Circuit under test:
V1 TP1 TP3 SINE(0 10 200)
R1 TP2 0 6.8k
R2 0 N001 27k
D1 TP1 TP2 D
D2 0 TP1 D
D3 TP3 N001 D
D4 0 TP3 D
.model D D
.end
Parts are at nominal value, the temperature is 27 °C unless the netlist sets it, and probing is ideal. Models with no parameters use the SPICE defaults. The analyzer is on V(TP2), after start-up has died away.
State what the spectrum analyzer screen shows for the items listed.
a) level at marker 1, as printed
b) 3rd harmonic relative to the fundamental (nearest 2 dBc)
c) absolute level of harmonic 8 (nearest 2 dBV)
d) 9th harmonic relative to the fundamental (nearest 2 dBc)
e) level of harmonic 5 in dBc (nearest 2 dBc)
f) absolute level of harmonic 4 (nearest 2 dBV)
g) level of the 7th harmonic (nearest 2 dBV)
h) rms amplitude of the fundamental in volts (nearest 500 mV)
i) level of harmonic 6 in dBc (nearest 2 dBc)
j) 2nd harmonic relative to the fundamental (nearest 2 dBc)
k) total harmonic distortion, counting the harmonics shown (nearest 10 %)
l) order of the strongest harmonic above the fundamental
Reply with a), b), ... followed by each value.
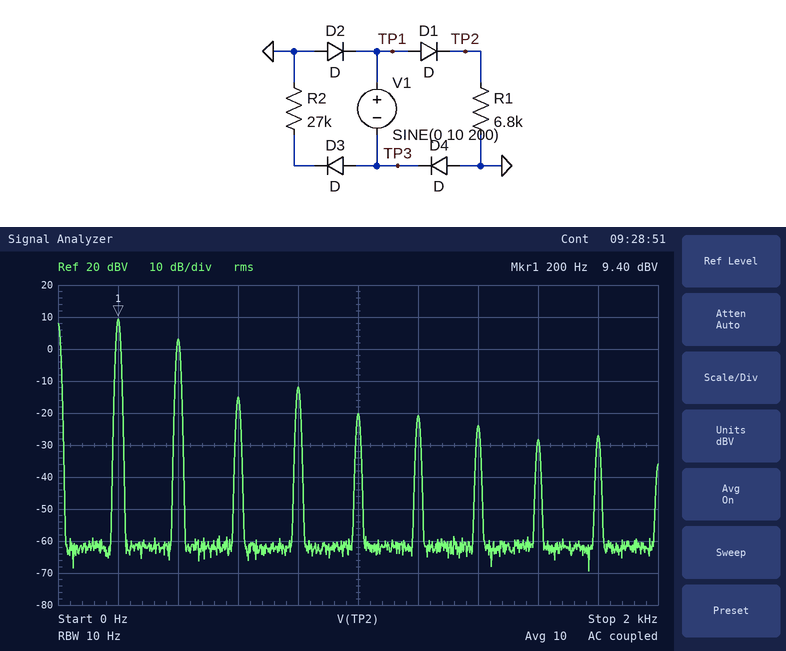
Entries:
a) 9.40 dBV
b) -24 dBc
c) -28 dBV
d) -36 dBc
e) -30 dBc
f) -12 dBV
g) -24 dBV
h) 3.0 V
i) -30 dBc
j) -6 dBc
k) 50 %
l) 2
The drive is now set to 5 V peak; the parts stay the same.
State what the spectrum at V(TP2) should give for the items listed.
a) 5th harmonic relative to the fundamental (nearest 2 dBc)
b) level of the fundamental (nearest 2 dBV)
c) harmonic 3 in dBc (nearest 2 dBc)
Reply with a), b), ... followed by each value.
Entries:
a) -24 dBc
b) 2 dBV
c) -18 dBc
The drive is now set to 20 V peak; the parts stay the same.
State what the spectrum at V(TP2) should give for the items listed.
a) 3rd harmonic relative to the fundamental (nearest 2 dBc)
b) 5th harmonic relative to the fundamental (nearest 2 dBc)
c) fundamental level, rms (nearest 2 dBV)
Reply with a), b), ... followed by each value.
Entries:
a) -30 dBc
b) -36 dBc
c) 16 dBV
